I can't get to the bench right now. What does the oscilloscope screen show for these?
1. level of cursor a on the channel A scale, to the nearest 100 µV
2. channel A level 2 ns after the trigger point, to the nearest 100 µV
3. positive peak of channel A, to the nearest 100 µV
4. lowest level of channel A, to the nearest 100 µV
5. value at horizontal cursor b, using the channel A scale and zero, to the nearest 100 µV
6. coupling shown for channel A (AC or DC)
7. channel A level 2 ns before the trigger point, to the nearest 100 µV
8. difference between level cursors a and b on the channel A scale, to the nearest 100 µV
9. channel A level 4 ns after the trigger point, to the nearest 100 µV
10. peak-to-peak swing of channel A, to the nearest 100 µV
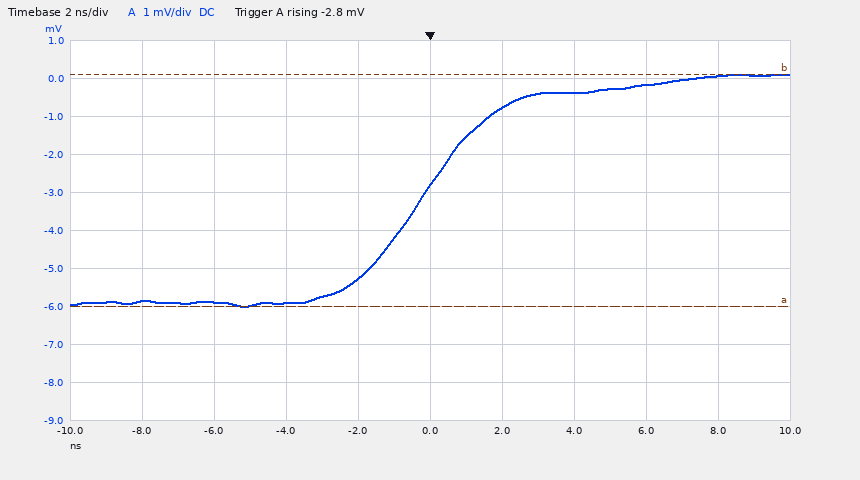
-6.0 mV
-800 µV
100 µV
-6.0 mV
100 µV
DC
-5.3 mV
6.1 mV
-400 µV
6.1 mV
